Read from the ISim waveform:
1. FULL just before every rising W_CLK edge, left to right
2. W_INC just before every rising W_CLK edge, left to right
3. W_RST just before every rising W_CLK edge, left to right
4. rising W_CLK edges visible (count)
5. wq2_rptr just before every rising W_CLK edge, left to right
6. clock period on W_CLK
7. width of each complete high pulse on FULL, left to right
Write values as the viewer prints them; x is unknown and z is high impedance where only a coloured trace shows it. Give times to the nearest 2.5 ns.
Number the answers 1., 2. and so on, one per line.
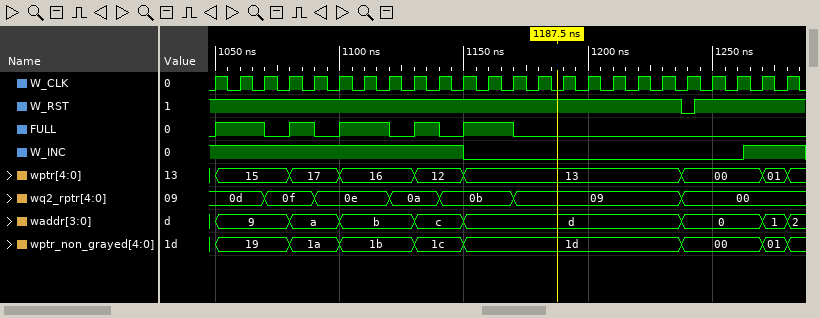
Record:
1. 0 1 1 0 1 0 1 1 0 1 0 1 1 0 0 0 0 0 0 0 0 0 0 0
2. 1 1 1 1 1 1 1 1 1 1 1 0 0 0 0 0 0 0 0 0 0 0 1 1
3. 1 1 1 1 1 1 1 1 1 1 1 1 1 1 1 1 1 1 1 0 1 1 1 1
4. 24
5. 0d, 0d, 0d, 0f, 0f, 0e, 0e, 0e, 0a, 0a, 0b, 0b, 0b, 09, 09, 09, 09, 09, 09, 00, 00, 00, 00, 00
6. 10 ns
7. 20 ns, 10 ns, 20 ns, 10 ns, 20 ns
